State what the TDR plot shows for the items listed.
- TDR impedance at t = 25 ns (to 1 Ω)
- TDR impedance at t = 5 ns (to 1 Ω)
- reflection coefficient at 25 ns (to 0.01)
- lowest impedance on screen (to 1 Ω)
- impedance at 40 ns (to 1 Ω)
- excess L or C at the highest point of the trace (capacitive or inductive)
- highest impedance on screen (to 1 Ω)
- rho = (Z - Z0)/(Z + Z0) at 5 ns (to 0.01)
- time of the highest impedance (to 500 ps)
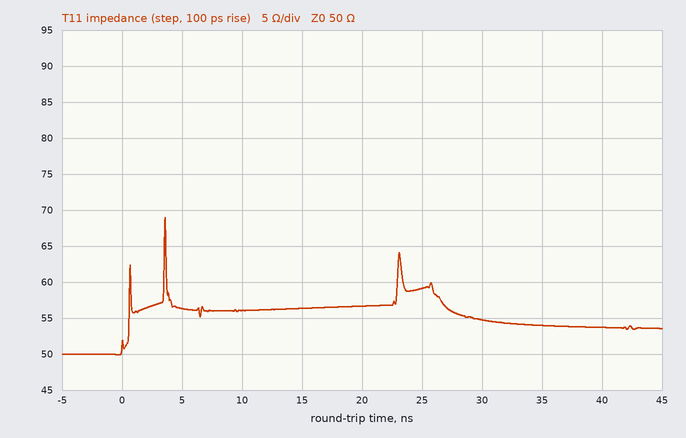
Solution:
59 Ω
56 Ω
+0.08
50 Ω
54 Ω
inductive
69 Ω
+0.06
3.5 ns
